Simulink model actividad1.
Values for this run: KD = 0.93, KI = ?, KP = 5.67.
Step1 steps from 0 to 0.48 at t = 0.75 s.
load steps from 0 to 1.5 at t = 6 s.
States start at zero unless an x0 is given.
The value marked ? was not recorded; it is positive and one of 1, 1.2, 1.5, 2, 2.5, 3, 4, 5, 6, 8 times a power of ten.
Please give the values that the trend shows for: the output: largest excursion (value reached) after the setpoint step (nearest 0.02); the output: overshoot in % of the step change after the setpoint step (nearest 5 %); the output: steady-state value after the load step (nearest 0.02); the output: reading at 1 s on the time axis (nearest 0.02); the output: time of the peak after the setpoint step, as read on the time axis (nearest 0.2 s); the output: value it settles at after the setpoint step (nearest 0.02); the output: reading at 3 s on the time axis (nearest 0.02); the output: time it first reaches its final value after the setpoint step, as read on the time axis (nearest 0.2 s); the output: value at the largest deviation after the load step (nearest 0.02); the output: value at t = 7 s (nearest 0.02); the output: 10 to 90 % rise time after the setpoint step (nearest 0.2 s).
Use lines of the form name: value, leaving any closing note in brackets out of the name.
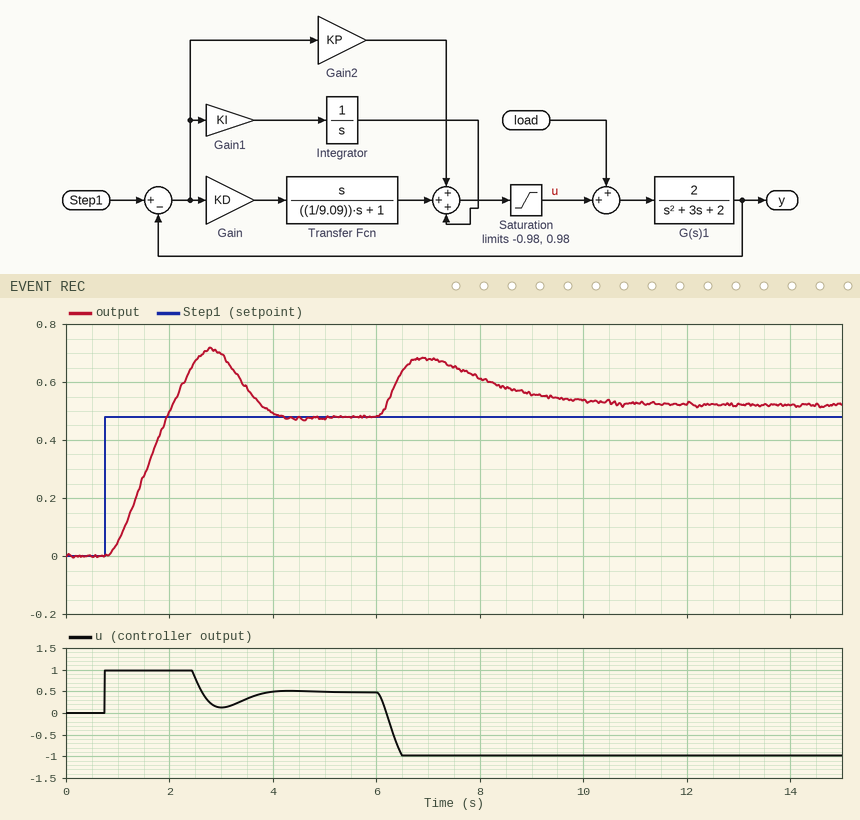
the output: largest excursion (value reached) after the setpoint step: 0.72
the output: overshoot in % of the step change after the setpoint step: 50 %
the output: steady-state value after the load step: 0.52
the output: reading at 1 s on the time axis: 0.04
the output: time of the peak after the setpoint step, as read on the time axis: 2.8 s
the output: value it settles at after the setpoint step: 0.48
the output: reading at 3 s on the time axis: 0.70
the output: time it first reaches its final value after the setpoint step, as read on the time axis: 2.0 s
the output: value at the largest deviation after the load step: 0.68
the output: value at t = 7 s: 0.68
the output: 10 to 90 % rise time after the setpoint step: 0.8 s
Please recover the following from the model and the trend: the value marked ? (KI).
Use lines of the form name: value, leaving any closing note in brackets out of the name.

the value marked ?: 8
